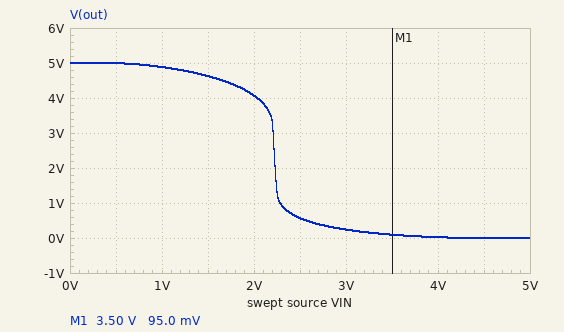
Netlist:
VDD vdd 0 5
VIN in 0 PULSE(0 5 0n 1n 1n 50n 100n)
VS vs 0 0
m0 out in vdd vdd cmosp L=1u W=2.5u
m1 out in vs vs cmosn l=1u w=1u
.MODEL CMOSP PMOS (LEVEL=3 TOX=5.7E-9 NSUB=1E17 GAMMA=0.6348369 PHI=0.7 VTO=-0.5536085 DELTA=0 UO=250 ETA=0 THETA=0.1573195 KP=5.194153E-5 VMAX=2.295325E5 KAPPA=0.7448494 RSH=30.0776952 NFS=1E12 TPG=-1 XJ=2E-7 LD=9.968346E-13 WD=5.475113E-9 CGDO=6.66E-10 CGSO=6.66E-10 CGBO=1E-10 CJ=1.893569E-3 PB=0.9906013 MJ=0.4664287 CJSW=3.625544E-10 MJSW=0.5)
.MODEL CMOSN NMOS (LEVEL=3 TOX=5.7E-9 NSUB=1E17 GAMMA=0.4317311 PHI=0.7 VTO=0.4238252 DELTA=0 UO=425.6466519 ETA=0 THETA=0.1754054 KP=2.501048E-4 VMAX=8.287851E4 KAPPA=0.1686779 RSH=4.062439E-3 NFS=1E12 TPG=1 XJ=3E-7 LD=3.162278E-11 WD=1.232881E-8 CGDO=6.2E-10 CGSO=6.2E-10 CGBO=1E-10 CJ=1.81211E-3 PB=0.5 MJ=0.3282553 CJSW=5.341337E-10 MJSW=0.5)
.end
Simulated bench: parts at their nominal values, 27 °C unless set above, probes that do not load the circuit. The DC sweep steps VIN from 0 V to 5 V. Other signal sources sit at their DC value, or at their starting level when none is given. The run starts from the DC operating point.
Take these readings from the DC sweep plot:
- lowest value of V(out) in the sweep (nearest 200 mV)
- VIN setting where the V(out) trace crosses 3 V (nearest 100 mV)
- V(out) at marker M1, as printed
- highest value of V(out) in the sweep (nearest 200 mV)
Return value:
0 V
2.2 V
95.0 mV
5.0 V
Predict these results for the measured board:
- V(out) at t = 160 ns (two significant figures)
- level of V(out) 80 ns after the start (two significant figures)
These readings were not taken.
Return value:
5.0 V
5.0 V
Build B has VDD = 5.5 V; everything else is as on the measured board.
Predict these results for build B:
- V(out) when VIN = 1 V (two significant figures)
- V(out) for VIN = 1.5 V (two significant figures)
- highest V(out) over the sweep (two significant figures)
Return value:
5.4 V
5.2 V
5.5 V
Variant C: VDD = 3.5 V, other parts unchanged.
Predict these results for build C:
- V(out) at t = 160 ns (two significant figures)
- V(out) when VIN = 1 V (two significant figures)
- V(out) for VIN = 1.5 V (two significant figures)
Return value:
3.5 V
3.3 V
2.6 V
